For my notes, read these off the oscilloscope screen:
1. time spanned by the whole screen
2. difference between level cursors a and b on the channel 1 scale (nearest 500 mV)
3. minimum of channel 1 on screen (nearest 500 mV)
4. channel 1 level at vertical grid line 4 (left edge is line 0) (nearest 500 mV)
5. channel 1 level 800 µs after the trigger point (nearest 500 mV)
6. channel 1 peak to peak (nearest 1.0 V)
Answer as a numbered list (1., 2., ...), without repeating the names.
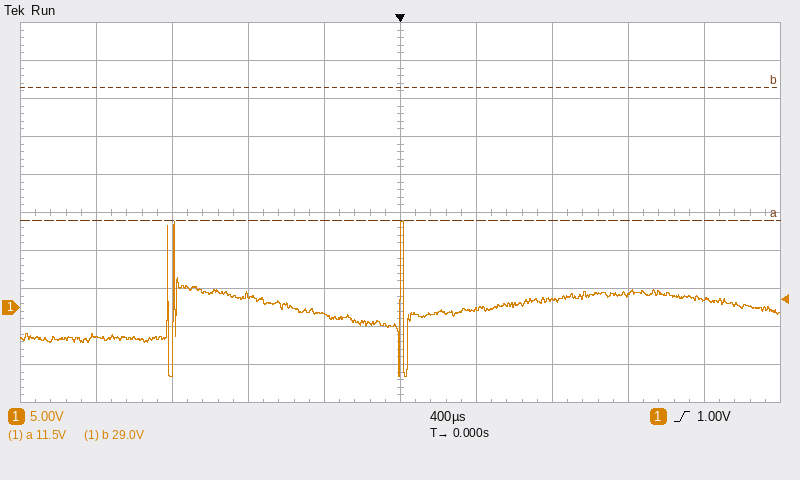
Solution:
1. 4 ms
2. 17.5 V
3. -9.0 V
4. -1.0 V
5. 1.0 V
6. 20.0 V
